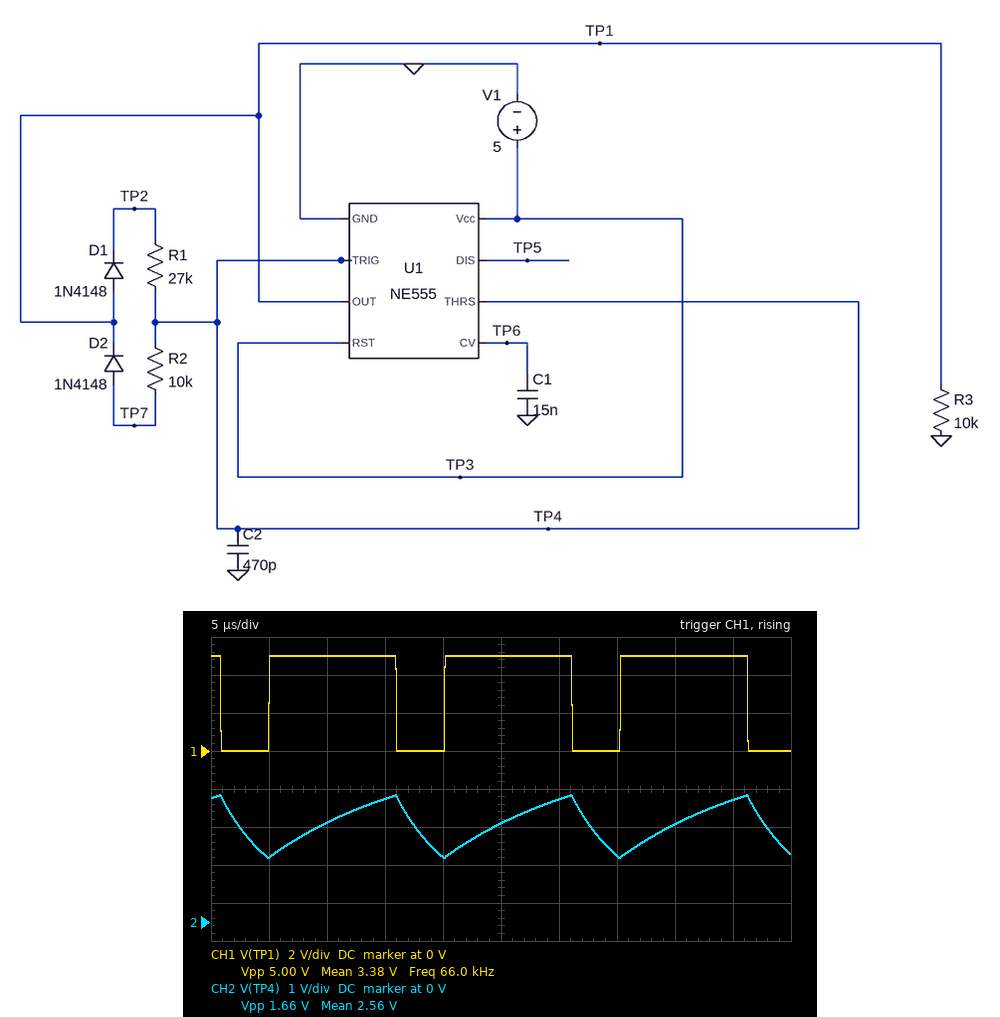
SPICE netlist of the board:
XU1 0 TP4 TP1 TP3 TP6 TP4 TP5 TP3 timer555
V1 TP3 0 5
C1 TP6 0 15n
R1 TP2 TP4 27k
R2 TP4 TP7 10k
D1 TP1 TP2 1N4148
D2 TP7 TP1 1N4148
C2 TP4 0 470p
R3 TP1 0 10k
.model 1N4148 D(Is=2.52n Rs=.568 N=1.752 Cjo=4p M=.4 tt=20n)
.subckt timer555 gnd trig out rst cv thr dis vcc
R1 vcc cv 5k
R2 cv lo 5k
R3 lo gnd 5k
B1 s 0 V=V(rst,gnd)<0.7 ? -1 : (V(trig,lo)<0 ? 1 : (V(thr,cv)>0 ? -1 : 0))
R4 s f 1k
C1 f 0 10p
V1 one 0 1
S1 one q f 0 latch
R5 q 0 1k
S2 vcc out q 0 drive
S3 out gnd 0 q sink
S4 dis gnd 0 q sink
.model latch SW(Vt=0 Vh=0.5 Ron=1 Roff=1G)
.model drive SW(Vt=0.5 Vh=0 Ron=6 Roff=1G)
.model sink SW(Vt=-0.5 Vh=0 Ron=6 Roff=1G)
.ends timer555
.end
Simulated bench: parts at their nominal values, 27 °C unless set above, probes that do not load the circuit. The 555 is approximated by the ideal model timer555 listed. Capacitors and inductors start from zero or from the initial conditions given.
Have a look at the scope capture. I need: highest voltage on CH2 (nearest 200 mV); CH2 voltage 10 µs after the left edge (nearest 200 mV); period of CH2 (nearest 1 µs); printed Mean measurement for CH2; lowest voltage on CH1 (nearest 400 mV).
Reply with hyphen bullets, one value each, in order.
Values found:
- 3.4 V
- 2.6 V
- 15 µs
- 2.56 V
- 0 V
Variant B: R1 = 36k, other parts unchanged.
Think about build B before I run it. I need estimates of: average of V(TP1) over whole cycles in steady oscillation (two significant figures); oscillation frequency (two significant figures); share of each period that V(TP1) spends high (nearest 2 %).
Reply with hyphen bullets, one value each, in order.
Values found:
- 3.9 V
- 54 kHz
- 78 %
